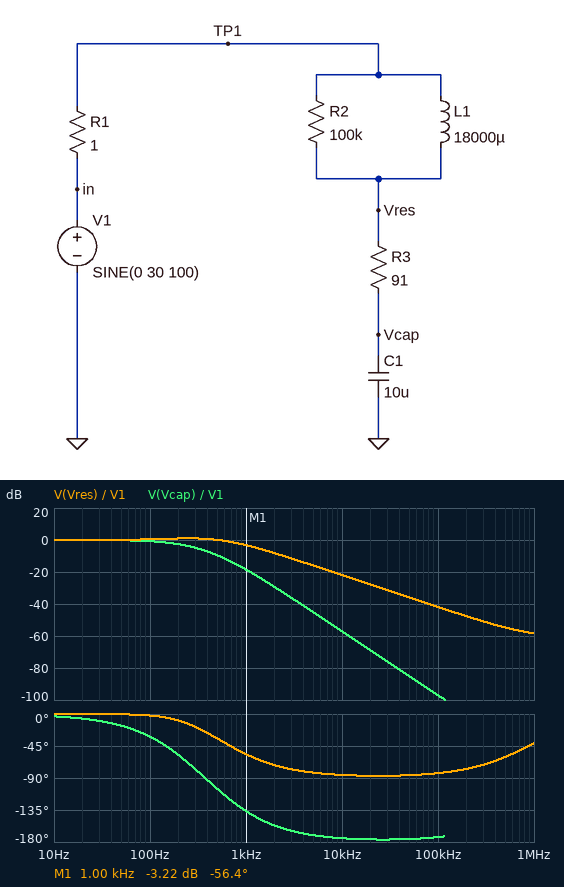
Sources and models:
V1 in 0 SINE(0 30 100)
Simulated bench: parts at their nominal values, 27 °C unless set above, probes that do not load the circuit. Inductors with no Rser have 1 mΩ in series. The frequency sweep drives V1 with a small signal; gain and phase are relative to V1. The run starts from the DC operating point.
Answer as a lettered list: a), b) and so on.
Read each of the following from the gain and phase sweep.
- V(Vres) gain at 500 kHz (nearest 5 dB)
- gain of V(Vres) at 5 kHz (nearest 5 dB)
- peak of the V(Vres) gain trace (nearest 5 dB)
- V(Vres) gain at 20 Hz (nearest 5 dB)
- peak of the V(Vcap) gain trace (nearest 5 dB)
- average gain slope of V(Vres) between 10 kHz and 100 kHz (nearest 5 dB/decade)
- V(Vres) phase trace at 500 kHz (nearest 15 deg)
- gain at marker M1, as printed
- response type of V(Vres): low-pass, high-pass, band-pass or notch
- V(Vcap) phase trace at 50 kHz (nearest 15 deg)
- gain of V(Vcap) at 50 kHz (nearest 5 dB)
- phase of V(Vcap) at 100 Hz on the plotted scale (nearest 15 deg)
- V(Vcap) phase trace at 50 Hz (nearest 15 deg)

a) -55 dB
b) -15 dB
c) 0 dB
d) 0 dB
e) 0 dB
f) -20 dB/decade
g) -60 deg
h) -3.22 dB
i) low-pass
j) -180 deg
k) -85 dB
l) -30 deg
m) -15 deg
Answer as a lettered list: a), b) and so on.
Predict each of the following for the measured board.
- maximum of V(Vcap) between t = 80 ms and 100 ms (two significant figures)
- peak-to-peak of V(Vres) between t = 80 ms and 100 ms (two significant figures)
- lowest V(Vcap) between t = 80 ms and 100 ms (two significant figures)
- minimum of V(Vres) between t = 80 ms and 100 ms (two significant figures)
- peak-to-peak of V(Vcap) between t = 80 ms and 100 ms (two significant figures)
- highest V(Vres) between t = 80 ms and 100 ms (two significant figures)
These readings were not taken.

a) 27 V
b) 63 V
c) -27 V
d) -32 V
e) 55 V
f) 32 V
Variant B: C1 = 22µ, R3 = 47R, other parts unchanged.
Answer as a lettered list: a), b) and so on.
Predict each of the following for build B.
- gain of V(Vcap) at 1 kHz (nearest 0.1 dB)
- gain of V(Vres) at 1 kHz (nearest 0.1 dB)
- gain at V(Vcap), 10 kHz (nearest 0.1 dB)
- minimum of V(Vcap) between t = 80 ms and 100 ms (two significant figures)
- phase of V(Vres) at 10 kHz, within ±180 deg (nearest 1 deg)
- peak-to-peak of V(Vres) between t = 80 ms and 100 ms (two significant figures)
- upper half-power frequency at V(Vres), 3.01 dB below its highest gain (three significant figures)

a) -24.1 dB
b) -7.8 dB
c) -63.9 dB
d) -28 V
e) -88 deg
f) 67 V
g) 447 Hz
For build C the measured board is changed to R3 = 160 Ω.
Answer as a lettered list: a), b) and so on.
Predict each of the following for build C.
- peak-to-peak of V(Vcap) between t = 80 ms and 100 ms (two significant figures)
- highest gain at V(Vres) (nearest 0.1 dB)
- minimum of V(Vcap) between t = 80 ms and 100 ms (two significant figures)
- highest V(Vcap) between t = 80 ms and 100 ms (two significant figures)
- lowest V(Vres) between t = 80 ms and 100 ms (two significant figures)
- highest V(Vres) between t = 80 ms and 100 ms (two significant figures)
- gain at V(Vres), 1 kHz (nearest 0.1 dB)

a) 44 V
b) 0.4 dB
c) -22 V
d) 22 V
e) -31 V
f) 31 V
g) -1.4 dB
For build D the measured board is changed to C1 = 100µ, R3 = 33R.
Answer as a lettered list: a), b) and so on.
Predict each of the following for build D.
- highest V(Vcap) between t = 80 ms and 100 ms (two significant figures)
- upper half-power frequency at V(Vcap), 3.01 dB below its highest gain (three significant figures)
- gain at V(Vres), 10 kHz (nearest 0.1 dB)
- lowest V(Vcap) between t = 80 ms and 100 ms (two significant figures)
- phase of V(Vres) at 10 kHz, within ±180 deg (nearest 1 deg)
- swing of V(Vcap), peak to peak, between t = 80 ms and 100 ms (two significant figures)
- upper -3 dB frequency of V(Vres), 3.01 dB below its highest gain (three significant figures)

a) 14 V
b) 55.1 Hz
c) -30.7 dB
d) -14 V
e) -88 deg
f) 28 V
g) 292 Hz
